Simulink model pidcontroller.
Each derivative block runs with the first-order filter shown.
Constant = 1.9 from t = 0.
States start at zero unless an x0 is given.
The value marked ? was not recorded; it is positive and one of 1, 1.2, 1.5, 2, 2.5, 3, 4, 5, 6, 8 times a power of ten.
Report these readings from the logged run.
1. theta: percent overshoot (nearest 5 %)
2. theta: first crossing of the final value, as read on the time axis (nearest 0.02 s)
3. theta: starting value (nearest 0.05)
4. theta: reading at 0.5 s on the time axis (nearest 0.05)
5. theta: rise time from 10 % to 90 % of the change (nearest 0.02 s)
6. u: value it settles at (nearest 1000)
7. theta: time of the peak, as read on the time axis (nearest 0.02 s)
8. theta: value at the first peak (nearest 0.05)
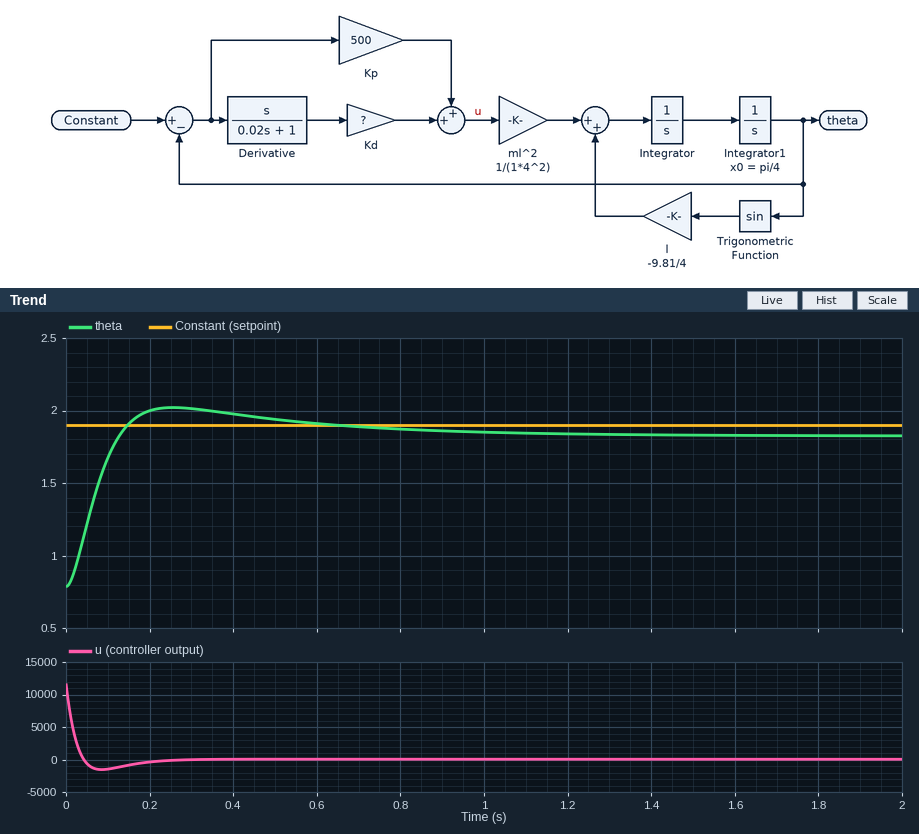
20 %
0.12 s
0.80
1.95
0.08 s
0
0.26 s
2.00
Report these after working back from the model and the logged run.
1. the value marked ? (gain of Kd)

200
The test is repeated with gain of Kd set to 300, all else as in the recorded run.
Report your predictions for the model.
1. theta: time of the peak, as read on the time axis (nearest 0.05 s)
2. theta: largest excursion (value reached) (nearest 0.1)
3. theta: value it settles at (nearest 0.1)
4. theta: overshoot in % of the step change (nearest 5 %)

0.15 s
2.0
1.8
15 %
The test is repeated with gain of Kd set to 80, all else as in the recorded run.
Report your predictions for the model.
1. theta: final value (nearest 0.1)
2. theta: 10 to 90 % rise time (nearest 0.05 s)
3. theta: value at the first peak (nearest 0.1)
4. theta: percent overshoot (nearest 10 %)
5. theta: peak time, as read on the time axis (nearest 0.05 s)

1.8
0.15 s
2.2
40 %
0.40 s
